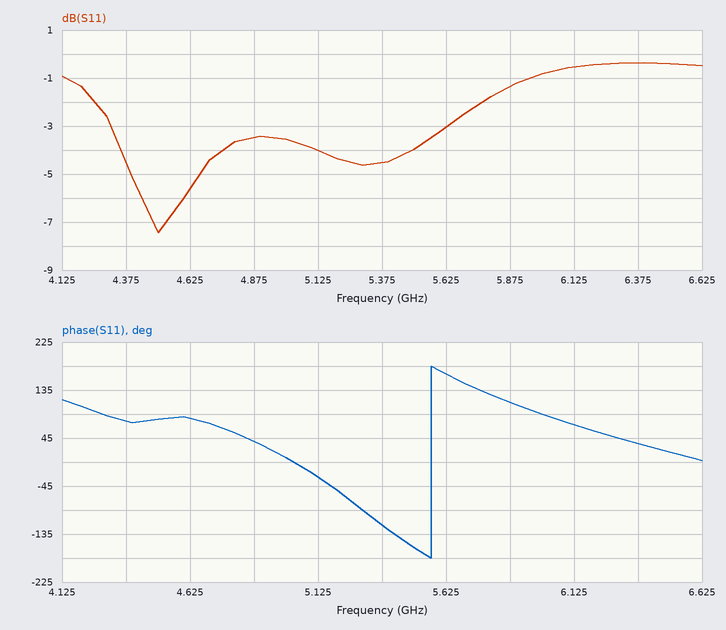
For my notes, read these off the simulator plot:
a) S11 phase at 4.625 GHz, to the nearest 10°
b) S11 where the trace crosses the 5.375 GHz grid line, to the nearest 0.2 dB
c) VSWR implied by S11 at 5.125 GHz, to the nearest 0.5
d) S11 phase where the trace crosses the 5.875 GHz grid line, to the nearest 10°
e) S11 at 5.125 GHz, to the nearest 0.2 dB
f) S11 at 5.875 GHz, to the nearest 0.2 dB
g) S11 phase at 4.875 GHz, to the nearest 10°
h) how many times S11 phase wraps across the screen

80°
-4.6 dB
4.5
110°
-4.0 dB
-1.4 dB
40°
1
